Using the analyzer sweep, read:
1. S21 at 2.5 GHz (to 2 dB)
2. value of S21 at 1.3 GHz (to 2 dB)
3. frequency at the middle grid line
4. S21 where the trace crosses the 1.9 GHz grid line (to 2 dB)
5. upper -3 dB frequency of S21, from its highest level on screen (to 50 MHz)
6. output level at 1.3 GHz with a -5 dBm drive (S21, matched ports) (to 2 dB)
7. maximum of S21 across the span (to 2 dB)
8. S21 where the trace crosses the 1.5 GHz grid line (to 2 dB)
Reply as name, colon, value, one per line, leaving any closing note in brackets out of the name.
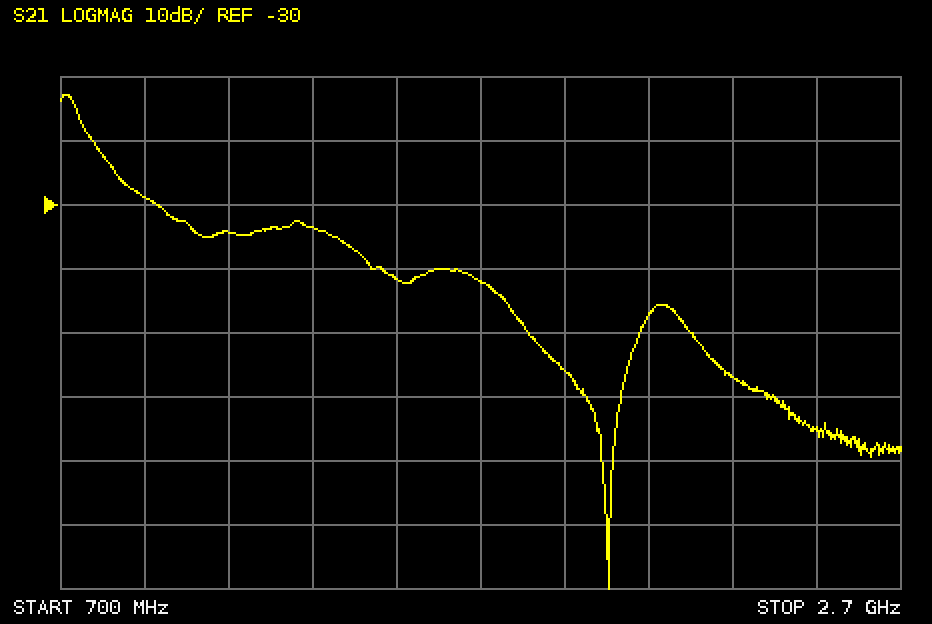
S21 at 2.5 GHz: -64 dB
value of S21 at 1.3 GHz: -34 dB
frequency at the middle grid line: 1.7 GHz
S21 where the trace crosses the 1.9 GHz grid line: -56 dB
upper -3 dB frequency of S21, from its highest level on screen: 750 MHz
output level at 1.3 GHz with a -5 dBm drive (S21, matched ports): -38 dBm
maximum of S21 across the span: -12 dB
S21 where the trace crosses the 1.5 GHz grid line: -42 dB
